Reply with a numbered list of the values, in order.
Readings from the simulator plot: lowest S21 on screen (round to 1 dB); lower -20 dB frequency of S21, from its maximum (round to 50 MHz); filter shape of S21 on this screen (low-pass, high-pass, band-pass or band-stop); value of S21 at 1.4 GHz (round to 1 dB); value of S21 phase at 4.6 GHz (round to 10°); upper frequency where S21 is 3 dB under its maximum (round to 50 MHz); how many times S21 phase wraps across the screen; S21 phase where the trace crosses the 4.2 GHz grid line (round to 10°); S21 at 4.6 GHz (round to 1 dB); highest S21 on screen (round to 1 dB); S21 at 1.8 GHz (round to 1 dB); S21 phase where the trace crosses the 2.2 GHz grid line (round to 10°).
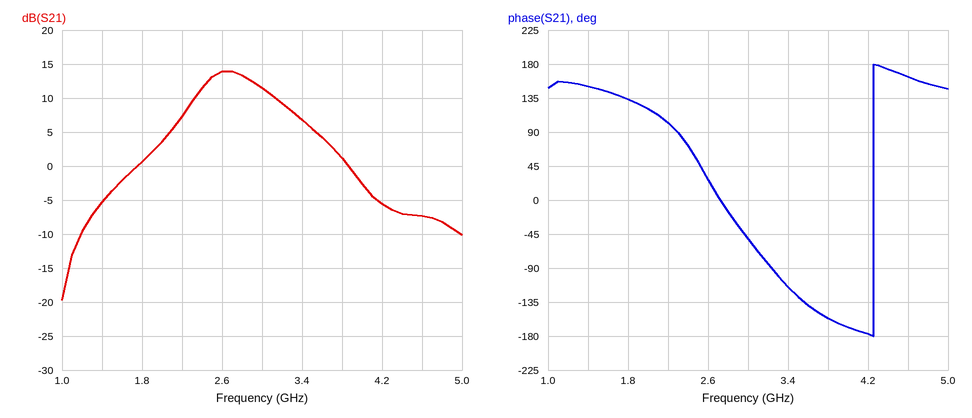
1. -20 dB
2. 1.35 GHz
3. band-pass
4. -5 dB
5. 160°
6. 3.05 GHz
7. 1
8. -180°
9. -7 dB
10. 14 dB
11. 1 dB
12. 100°
